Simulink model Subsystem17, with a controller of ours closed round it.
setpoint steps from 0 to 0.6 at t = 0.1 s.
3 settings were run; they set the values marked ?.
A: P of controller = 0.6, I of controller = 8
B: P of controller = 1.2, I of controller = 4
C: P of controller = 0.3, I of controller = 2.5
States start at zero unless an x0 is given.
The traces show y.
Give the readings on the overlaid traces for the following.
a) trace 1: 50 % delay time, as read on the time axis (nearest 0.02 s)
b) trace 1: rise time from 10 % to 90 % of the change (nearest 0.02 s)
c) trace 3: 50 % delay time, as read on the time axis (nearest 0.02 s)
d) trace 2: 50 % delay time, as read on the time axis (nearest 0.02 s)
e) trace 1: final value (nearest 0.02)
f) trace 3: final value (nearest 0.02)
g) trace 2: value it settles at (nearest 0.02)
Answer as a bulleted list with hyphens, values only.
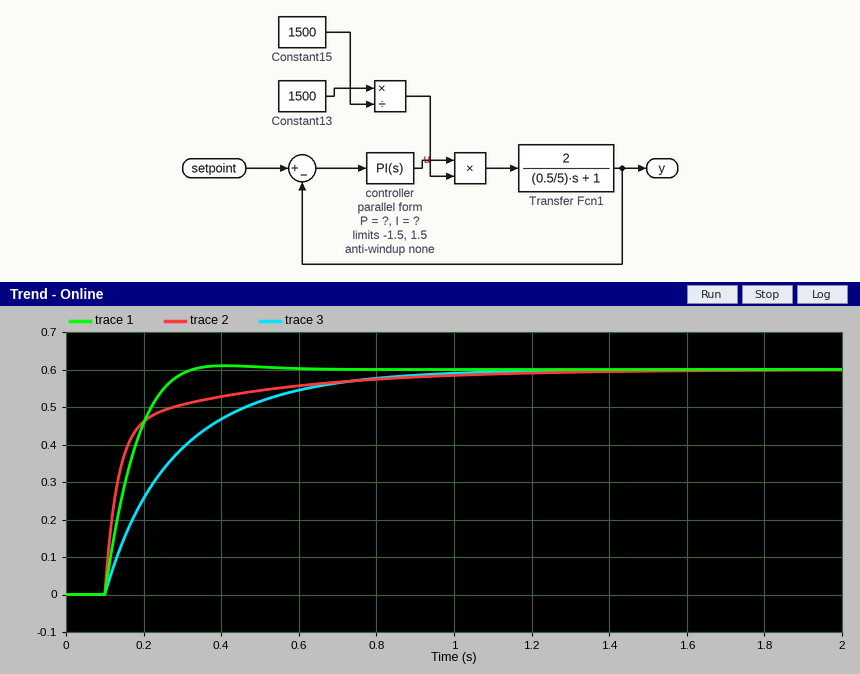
- 0.16 s
- 0.14 s
- 0.22 s
- 0.14 s
- 0.60
- 0.60
- 0.60
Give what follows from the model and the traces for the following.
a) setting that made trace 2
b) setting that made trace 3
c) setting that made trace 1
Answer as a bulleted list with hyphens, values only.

- B
- C
- A
